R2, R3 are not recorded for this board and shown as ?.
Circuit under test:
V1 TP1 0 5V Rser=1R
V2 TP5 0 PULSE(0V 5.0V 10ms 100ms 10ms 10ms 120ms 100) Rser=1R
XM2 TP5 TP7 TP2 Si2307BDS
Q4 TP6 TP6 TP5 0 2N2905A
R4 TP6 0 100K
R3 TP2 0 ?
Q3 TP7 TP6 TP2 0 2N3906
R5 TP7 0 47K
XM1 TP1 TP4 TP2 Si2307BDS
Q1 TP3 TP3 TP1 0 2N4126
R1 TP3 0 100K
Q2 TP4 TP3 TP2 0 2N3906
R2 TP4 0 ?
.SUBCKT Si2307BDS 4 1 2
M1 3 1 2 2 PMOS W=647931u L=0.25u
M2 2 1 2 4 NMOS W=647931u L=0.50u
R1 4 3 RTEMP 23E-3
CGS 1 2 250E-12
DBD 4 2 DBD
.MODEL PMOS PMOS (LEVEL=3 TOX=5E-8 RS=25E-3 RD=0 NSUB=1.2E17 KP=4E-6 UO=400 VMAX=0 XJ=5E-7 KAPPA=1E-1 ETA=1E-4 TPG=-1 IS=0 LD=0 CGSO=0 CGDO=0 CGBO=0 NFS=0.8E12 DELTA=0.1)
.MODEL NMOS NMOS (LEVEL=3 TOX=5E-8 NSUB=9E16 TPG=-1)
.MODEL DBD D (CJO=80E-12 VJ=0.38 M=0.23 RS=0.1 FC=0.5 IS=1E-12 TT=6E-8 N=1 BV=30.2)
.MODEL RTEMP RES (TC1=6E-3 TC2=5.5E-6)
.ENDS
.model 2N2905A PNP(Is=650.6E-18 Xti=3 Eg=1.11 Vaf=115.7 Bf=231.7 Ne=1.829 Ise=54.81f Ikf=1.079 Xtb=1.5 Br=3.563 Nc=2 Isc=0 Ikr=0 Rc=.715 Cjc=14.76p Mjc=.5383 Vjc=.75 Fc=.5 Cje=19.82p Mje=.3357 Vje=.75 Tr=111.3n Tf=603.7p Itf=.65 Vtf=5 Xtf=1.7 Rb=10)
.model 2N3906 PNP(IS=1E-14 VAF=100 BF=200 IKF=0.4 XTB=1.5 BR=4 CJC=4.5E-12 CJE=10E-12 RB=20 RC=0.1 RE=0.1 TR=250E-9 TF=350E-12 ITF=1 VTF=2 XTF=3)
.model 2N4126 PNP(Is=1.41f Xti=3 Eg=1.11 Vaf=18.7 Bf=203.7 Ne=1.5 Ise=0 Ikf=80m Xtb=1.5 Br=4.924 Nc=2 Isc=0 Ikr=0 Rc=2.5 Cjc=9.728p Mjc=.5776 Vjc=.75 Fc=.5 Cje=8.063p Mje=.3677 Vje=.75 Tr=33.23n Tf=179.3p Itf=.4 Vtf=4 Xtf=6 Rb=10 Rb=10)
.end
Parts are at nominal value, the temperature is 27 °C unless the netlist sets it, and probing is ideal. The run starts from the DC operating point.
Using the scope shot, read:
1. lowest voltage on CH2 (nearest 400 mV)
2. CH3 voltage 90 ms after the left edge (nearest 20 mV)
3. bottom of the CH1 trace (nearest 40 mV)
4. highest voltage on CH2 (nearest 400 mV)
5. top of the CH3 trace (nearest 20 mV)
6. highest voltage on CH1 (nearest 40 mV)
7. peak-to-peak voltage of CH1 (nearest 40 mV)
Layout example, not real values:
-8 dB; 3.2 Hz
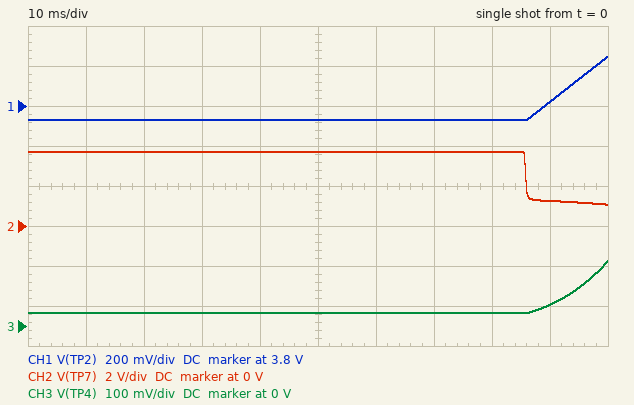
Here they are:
1.2 V; 60 mV; 3.72 V; 3.6 V; 160 mV; 4.04 V; 320 mV
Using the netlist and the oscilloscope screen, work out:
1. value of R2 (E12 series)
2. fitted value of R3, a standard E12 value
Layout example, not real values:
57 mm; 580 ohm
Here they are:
27 kΩ; 3.3 Ω
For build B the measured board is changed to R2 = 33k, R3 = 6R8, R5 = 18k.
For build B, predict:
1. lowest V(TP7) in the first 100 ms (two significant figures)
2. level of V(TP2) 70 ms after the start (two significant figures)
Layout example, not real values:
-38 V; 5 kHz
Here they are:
1.7 V; 4.3 V
